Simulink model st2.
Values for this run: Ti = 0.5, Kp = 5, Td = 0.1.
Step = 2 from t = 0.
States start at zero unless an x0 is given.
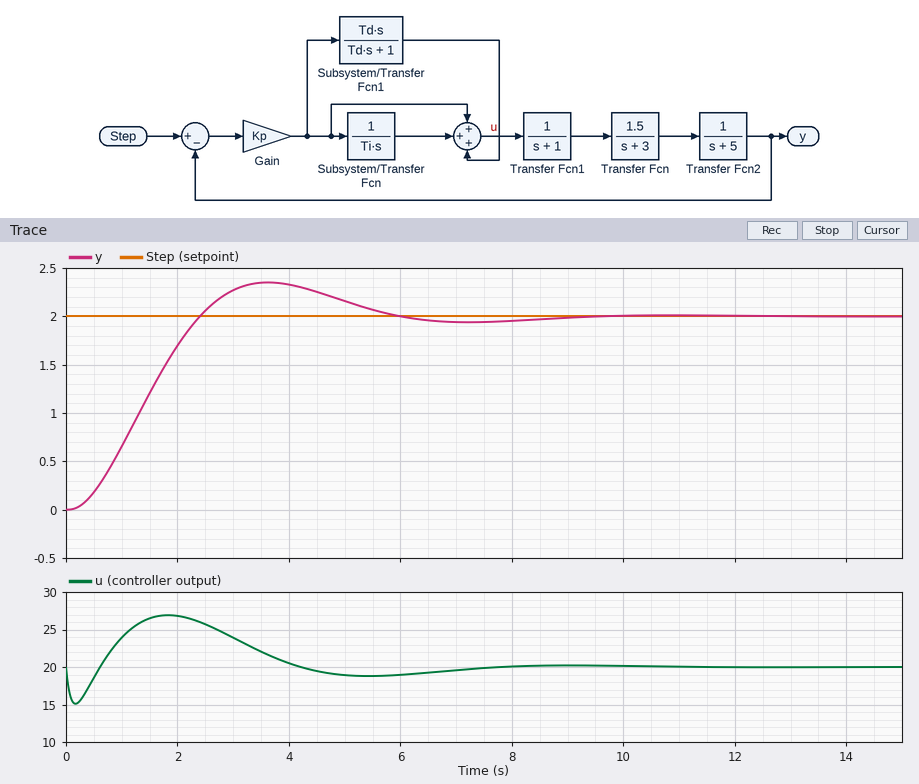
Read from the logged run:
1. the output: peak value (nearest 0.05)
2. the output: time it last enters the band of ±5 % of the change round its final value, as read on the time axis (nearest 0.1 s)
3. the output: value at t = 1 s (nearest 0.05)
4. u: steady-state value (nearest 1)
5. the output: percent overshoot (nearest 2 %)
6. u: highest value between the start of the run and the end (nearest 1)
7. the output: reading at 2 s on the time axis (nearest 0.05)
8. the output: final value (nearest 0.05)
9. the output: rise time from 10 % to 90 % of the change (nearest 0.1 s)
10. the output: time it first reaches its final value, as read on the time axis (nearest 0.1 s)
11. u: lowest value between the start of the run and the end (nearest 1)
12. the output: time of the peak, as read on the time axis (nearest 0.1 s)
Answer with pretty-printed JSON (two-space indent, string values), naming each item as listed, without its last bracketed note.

{
  "the output: peak value": "2.35",
  "the output: time it last enters the band of ±5 % of the change round its final value, as read on the time axis": "5.3 s",
  "the output: value at t = 1 s": "0.65",
  "u: steady-state value": "20",
  "the output: percent overshoot": "18 %",
  "u: highest value between the start of the run and the end": "27",
  "the output: reading at 2 s on the time axis": "1.70",
  "the output: final value": "2.00",
  "the output: rise time from 10 % to 90 % of the change": "1.6 s",
  "the output: time it first reaches its final value, as read on the time axis": "2.4 s",
  "u: lowest value between the start of the run and the end": "15",
  "the output: time of the peak, as read on the time axis": "3.6 s"
}
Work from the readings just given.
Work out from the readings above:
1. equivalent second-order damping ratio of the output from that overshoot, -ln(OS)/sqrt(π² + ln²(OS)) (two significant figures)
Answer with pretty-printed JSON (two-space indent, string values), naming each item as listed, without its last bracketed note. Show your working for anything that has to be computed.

{
  "equivalent second-order damping ratio of the output from that overshoot, -ln(OS)/sqrt(π² + ln²(OS))": "ln(0.18) = -1.715; 1.715 / sqrt(9.870 + 2.941) = 0.48"
}
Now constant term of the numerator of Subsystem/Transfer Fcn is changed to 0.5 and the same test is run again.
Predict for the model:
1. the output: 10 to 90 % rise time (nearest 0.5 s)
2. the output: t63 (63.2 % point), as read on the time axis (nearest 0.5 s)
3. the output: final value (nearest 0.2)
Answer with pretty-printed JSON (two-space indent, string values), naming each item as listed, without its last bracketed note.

{
  "the output: 10 to 90 % rise time": "3.5 s",
  "the output: t63 (63.2 % point), as read on the time axis": "2.0 s",
  "the output: final value": "2.0"
}
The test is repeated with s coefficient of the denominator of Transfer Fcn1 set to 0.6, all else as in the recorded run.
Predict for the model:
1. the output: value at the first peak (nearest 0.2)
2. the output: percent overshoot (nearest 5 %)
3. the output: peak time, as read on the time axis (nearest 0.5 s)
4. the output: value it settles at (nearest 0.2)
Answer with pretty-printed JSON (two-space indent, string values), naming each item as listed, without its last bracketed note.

{
  "the output: value at the first peak": "2.2",
  "the output: percent overshoot": "10 %",
  "the output: peak time, as read on the time axis": "3.0 s",
  "the output: value it settles at": "2.0"
}
